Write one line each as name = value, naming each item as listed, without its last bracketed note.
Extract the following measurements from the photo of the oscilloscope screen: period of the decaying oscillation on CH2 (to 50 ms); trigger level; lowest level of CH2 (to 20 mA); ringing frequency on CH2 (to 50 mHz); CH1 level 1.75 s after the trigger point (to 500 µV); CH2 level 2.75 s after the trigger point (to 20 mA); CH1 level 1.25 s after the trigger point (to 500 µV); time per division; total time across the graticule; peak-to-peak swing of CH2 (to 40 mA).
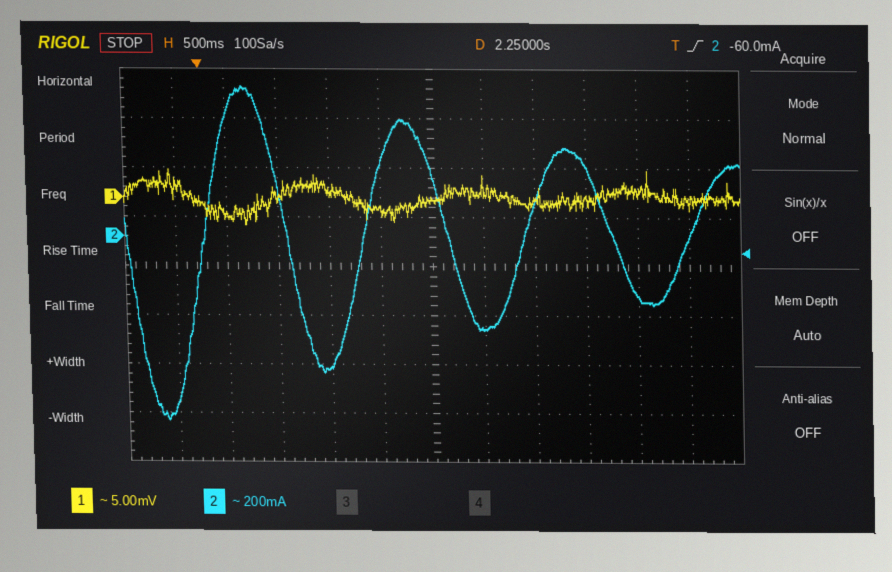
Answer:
period of the decaying oscillation on CH2 = 1.55 s
trigger level = -60.0 mA
lowest level of CH2 = -740 mA
ringing frequency on CH2 = 650 mHz
CH1 level 1.75 s after the trigger point = -1.5 mV
CH2 level 2.75 s after the trigger point = -380 mA
CH1 level 1.25 s after the trigger point = 500 µV
time per division = 500 ms
total time across the graticule = 6 s
peak-to-peak swing of CH2 = 1.36 A
